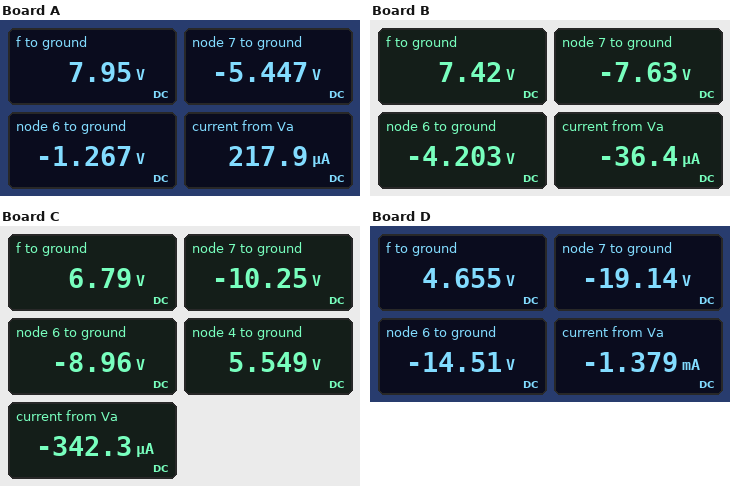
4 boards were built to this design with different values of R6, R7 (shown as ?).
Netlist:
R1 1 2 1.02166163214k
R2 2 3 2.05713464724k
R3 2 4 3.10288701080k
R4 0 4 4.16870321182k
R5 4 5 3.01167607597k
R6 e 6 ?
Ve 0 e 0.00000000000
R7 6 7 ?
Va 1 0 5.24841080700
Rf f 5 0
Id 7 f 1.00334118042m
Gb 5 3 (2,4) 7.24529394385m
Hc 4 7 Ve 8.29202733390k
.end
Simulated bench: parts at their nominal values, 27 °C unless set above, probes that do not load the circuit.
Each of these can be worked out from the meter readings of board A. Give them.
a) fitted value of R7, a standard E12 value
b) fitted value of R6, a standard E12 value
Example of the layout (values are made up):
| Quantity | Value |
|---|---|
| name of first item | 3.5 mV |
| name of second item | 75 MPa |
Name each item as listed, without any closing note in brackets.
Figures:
| Quantity | Value |
|---|---|
| fitted value of R7, a standard E12 value | 3.3 kΩ |
| fitted value of R6, a standard E12 value | 1 kΩ |
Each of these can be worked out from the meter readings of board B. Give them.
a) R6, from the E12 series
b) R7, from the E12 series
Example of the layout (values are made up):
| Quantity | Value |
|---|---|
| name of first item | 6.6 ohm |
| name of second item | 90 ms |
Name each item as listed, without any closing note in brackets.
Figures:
| Quantity | Value |
|---|---|
| R6, from the E12 series | 2.7 kΩ |
| R7, from the E12 series | 2.2 kΩ |
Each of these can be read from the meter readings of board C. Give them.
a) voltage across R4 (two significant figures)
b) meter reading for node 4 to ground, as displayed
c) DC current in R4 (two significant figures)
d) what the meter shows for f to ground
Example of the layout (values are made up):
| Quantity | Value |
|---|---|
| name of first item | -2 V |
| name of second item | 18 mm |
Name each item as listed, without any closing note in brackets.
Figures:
| Quantity | Value |
|---|---|
| voltage across R4 | 5.5 V |
| meter reading for node 4 to ground, as displayed | 5.549 V |
| DC current in R4 | 1.3 mA |
| what the meter shows for f to ground | 6.79 V |
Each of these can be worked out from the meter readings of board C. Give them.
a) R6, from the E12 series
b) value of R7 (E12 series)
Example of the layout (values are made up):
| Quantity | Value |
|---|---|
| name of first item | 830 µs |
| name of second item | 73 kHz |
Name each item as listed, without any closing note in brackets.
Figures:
| Quantity | Value |
|---|---|
| R6, from the E12 series | 4.7 kΩ |
| value of R7 | 680 Ω |
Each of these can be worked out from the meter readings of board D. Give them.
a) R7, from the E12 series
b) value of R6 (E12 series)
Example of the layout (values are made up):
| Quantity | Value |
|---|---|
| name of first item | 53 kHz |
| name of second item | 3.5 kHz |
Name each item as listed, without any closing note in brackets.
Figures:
| Quantity | Value |
|---|---|
| R7, from the E12 series | 1.5 kΩ |
| value of R6 | 4.7 kΩ |
